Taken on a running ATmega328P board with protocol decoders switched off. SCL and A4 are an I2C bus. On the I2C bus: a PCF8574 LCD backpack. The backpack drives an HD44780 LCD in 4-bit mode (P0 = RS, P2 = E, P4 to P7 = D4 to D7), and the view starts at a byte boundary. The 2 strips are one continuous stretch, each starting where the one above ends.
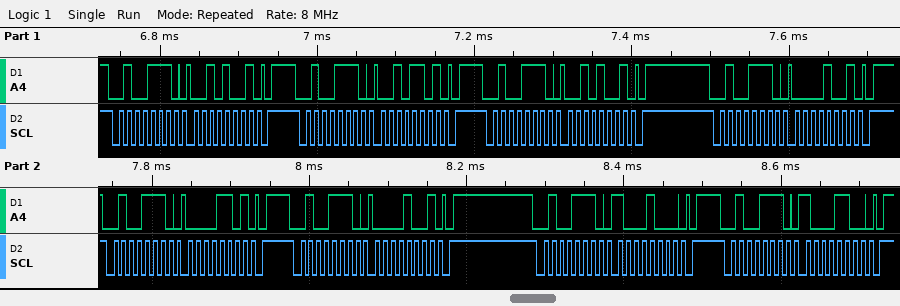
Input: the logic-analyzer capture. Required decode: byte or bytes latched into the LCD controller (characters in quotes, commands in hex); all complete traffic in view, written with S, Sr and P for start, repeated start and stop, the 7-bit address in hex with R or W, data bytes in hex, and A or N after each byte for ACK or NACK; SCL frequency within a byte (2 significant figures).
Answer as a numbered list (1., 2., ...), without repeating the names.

1. ' '
2. S 27W A 29 A P S 27W A 2D A P S 27W A 29 A P S 27W A 09 A P S 27W A 0D A P S 27W A 09 A P S 27W A 88 A P S 27W A 8C A P
3. 100 kHz
